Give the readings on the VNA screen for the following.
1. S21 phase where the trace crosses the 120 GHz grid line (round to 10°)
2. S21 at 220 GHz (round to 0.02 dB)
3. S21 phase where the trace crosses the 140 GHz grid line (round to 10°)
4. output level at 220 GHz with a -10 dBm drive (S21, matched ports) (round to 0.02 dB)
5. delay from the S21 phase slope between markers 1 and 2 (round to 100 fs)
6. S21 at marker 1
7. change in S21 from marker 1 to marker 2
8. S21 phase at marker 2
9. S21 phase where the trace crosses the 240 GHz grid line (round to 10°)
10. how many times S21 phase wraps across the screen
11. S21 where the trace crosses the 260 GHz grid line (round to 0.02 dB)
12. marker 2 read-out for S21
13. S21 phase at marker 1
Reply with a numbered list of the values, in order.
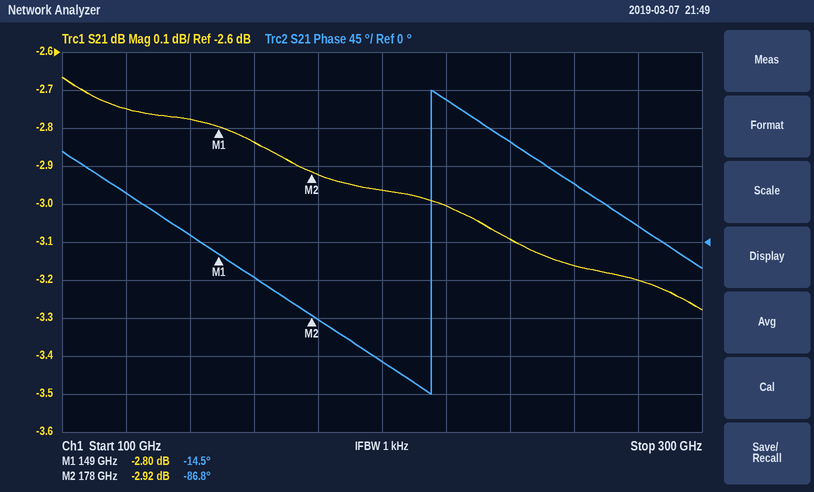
1. 60°
2. -3.00 dB
3. 10°
4. -13.00 dBm
5. 6.9 ps
6. -2.80 dB
7. -0.12 dB
8. -86.8°
9. 120°
10. 1
11. -3.16 dB
12. -2.92 dB
13. -14.5°
